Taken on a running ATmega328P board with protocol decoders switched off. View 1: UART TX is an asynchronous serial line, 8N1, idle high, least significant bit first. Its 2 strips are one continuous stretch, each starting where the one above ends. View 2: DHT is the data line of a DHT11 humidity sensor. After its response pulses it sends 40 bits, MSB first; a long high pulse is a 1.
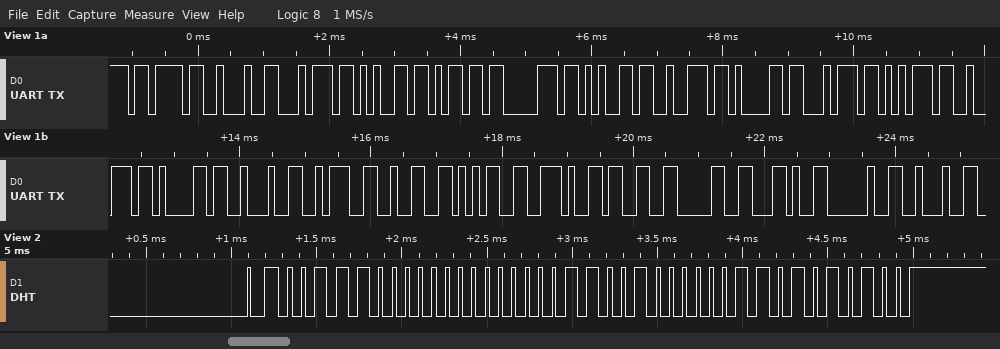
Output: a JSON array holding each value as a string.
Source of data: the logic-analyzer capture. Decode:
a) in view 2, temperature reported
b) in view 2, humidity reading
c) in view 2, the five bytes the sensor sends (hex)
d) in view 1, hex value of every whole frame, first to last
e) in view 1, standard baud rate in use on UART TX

["25.3 °C", "56 %", "38 00 19 03 54", "7B 22 74 65 6D 70 65 72 61 74 75 72 61 22 3A 32 35 2E 33 30 2C 20 22", "9600 baud"]
